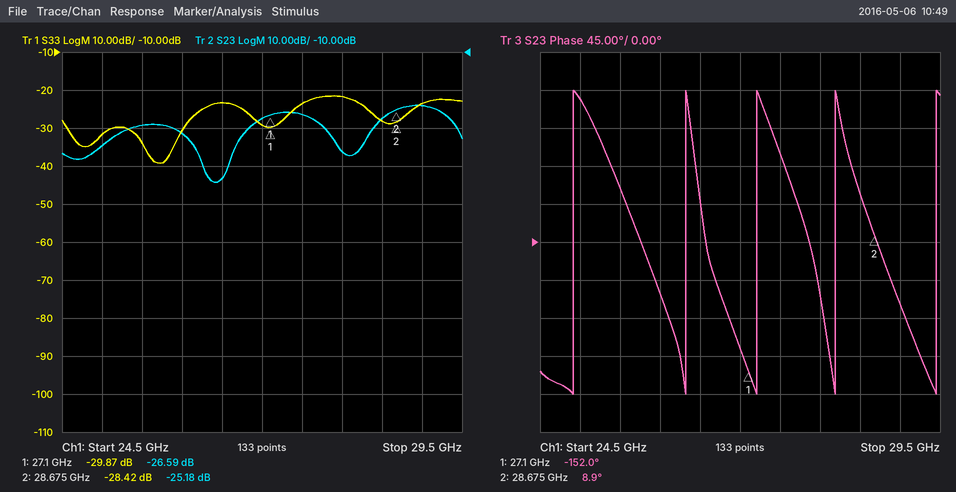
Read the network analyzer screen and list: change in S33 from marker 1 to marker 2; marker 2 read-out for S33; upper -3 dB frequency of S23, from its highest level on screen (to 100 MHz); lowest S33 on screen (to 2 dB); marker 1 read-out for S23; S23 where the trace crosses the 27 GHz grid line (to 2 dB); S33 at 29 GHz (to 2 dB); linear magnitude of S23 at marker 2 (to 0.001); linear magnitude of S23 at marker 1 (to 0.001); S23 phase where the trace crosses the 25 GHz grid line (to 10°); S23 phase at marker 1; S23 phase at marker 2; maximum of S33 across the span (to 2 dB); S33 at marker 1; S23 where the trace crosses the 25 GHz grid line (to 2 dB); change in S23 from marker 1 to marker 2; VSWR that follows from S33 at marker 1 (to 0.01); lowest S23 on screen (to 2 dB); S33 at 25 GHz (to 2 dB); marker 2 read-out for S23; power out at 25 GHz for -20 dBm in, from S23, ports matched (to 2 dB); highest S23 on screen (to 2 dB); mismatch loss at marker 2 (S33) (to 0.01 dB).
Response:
1.45 dB
-28.42 dB
29.3 GHz
-40 dB
-26.59 dB
-28 dB
-24 dB
0.055
0.047
170°
-152.0°
8.9°
-22 dB
-29.87 dB
-34 dB
1.41 dB
1.07
-44 dB
-32 dB
-25.18 dB
-54 dBm
-24 dB
0.01 dB
